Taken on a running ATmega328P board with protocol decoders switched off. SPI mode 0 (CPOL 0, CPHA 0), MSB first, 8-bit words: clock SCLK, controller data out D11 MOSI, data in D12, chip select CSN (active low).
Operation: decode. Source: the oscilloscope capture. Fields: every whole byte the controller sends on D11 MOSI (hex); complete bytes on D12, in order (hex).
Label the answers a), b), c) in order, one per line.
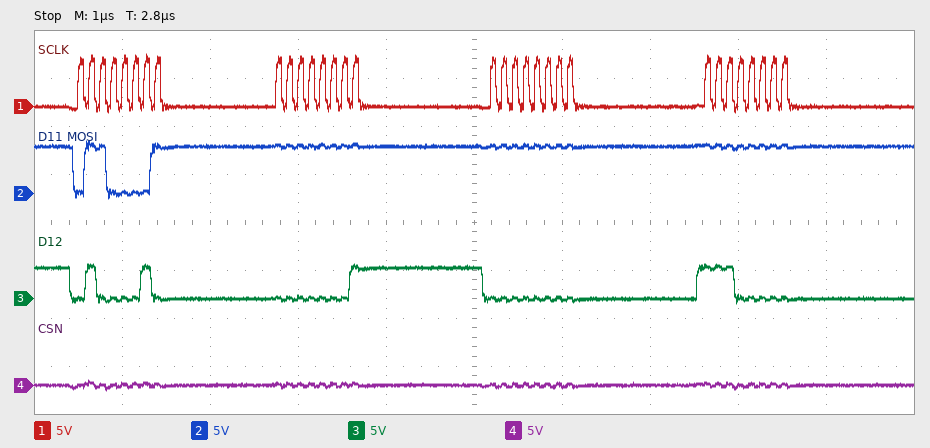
a) 61 FF FF FF
b) 42 01 00 E0
